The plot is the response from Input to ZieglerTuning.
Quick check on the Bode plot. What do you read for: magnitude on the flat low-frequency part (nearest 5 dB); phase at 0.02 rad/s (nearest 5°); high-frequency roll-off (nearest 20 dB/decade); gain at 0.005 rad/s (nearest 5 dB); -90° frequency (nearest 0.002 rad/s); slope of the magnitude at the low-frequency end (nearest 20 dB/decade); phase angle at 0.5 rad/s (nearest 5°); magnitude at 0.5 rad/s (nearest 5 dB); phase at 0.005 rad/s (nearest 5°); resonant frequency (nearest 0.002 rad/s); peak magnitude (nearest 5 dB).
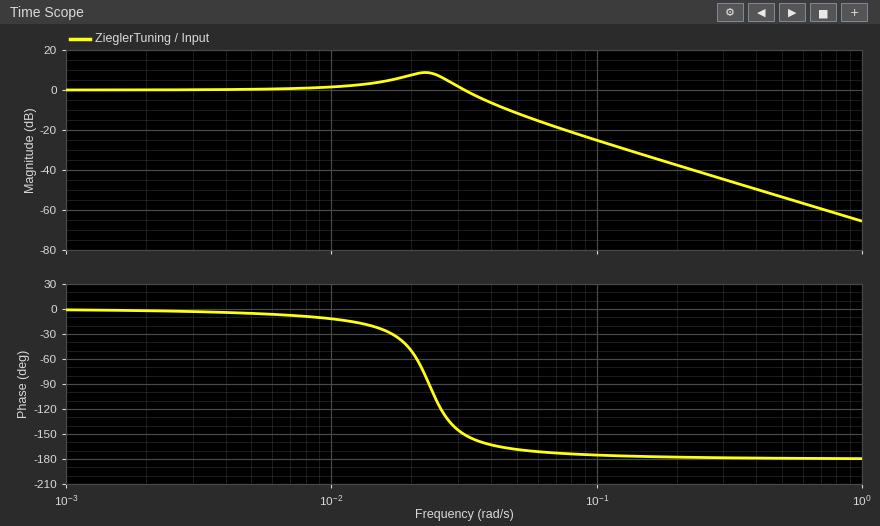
0 dB
-50°
-40 dB/decade
0 dB
0.024 rad/s
0 dB/decade
-180°
-55 dB
-5°
0.022 rad/s
10 dB
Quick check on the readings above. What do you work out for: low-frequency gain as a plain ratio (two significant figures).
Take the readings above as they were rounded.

1.0
